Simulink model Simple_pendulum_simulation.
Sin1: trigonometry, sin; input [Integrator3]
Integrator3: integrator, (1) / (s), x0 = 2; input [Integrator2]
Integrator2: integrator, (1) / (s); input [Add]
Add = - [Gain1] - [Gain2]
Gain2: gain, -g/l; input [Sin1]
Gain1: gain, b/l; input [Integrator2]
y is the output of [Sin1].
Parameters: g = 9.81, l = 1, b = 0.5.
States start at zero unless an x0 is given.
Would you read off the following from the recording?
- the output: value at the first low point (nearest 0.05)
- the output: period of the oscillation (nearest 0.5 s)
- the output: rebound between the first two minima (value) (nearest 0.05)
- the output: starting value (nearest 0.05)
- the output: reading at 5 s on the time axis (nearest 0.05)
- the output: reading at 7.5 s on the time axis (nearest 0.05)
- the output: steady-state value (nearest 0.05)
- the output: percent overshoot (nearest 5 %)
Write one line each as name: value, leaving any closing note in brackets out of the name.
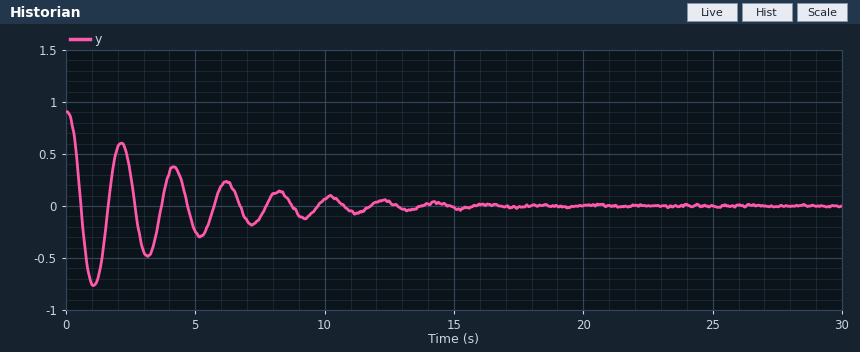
the output: value at the first low point: -0.75
the output: period of the oscillation: 2.0 s
the output: rebound between the first two minima (value): 0.60
the output: starting value: 0.90
the output: reading at 5 s on the time axis: -0.25
the output: reading at 7.5 s on the time axis: -0.10
the output: steady-state value: 0.00
the output: percent overshoot: 85 %
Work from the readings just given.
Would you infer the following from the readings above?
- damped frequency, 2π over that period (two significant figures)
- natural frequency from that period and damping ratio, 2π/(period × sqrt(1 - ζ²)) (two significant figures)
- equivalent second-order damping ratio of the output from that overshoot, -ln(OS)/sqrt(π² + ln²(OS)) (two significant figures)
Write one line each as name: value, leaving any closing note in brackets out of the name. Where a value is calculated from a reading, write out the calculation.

damped frequency, 2π over that period: 2π / 2 = 3.1 rad/s
natural frequency from that period and damping ratio, 2π/(period × sqrt(1 - ζ²)): 2π / (2 × sqrt(1 - 0.052²)) = 3.1 rad/s
equivalent second-order damping ratio of the output from that overshoot, -ln(OS)/sqrt(π² + ln²(OS)): ln(0.85) = -0.163; 0.163 / sqrt(9.870 + 0.026) = 0.052
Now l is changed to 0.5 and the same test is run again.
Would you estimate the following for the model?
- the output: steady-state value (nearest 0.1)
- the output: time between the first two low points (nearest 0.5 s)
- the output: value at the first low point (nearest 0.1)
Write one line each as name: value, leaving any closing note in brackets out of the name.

the output: steady-state value: 0.0
the output: time between the first two low points: 1.5 s
the output: value at the first low point: -0.7
